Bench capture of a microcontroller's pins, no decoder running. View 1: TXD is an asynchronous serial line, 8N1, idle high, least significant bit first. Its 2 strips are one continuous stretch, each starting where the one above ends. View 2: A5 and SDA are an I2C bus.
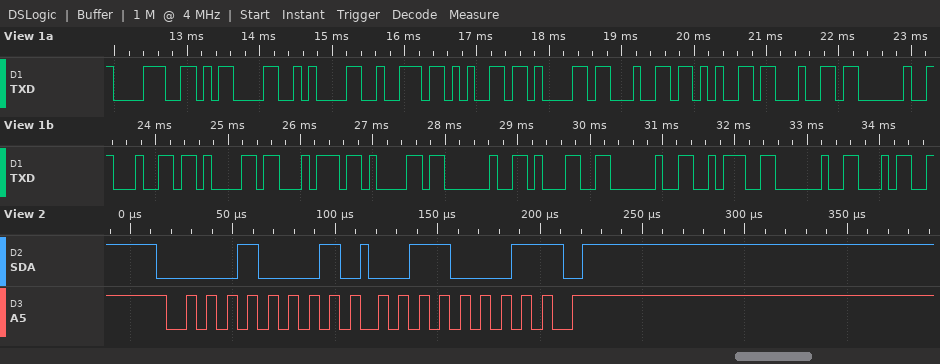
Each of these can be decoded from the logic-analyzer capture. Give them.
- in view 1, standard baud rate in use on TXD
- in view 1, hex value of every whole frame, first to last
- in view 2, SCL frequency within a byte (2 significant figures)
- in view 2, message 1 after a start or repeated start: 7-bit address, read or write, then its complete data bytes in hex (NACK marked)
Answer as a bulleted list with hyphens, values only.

- 9600 baud
- 38 0D 0A 72 65 61 64 65 64 20 64 61 74 61 20 31 20 3A 20 34
- 100 kHz
- 0x08 read: 31 NACK
